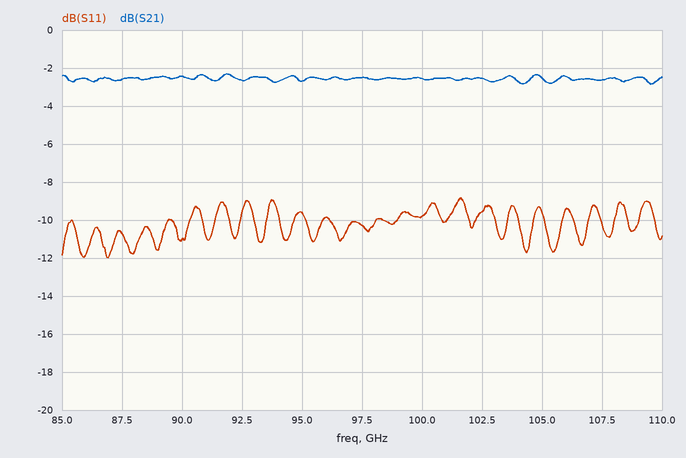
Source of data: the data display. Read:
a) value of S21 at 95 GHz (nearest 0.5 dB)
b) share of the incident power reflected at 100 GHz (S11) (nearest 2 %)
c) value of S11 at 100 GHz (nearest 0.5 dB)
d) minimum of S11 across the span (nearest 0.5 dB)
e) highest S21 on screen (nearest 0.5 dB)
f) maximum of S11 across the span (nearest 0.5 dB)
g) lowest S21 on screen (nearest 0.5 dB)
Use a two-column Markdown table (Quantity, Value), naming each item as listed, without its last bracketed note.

| Quantity | Value |
|---|---|
| value of S21 at 95 GHz | -2.5 dB |
| share of the incident power reflected at 100 GHz (S11) | 10 % |
| value of S11 at 100 GHz | -10.0 dB |
| minimum of S11 across the span | -12.0 dB |
| highest S21 on screen | -2.5 dB |
| maximum of S11 across the span | -9.0 dB |
| lowest S21 on screen | -3.0 dB |
